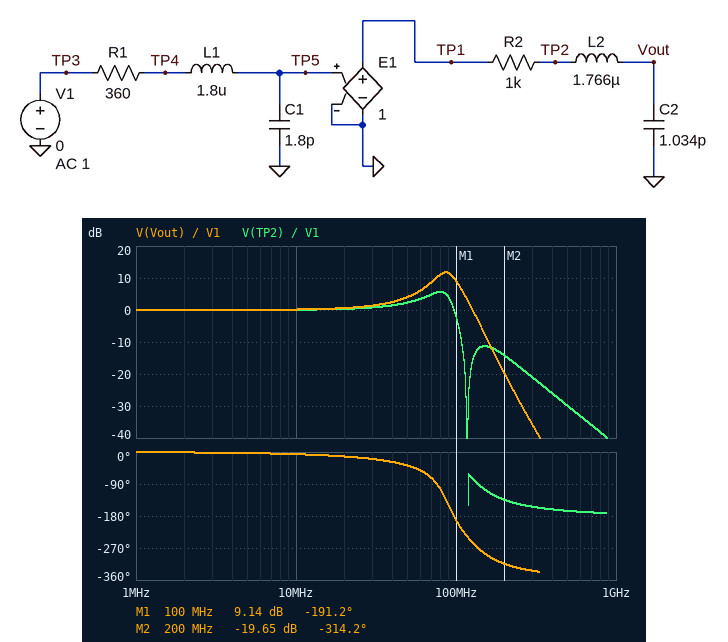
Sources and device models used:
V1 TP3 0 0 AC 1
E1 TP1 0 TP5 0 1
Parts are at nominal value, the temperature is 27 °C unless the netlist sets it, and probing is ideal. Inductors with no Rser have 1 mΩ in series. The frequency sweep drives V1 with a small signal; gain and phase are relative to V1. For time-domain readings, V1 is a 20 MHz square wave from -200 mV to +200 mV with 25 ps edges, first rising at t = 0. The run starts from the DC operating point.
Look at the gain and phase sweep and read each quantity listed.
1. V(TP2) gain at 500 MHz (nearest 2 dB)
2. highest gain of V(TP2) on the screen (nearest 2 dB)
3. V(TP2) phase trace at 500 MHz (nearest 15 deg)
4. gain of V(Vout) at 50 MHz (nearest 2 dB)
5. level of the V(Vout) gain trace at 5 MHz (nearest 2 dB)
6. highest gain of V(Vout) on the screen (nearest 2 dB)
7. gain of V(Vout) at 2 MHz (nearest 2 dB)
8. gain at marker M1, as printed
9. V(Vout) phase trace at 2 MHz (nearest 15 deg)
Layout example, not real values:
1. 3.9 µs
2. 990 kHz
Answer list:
1. -30 dB
2. 6 dB
3. -165 deg
4. 4 dB
5. 0 dB
6. 12 dB
7. 0 dB
8. 9.14 dB
9. 0 deg
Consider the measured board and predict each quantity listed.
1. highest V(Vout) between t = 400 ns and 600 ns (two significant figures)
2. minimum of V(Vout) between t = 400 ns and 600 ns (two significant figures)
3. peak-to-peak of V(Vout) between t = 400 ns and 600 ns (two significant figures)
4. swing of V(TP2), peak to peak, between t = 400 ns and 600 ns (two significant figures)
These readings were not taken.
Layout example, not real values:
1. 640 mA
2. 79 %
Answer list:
1. 510 mV
2. -510 mV
3. 1.0 V
4. 670 mV
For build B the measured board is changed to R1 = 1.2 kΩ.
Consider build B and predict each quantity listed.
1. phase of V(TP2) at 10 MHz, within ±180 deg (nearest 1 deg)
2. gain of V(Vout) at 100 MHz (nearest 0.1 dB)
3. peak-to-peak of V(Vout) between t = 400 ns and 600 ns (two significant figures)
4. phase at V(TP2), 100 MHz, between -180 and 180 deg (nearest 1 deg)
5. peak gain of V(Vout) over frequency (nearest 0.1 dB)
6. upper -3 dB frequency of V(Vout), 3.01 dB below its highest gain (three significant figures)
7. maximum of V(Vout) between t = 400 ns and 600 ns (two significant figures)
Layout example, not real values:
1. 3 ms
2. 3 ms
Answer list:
1. -12 deg
2. 0.2 dB
3. 600 mV
4. -168 deg
5. 1.9 dB
6. 109 MHz
7. 300 mV
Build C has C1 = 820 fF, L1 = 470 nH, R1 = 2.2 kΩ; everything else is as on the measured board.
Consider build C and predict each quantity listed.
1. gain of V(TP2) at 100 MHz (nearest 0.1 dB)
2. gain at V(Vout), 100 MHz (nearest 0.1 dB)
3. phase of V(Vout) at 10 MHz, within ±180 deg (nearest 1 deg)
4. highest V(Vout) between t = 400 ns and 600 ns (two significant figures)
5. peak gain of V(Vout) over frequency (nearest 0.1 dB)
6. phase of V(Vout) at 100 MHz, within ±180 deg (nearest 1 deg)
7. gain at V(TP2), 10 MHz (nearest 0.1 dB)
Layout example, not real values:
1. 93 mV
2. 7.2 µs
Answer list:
1. -11.1 dB
2. 0 dB
3. -10 deg
4. 250 mV
5. 0.4 dB
6. -120 deg
7. -0.1 dB
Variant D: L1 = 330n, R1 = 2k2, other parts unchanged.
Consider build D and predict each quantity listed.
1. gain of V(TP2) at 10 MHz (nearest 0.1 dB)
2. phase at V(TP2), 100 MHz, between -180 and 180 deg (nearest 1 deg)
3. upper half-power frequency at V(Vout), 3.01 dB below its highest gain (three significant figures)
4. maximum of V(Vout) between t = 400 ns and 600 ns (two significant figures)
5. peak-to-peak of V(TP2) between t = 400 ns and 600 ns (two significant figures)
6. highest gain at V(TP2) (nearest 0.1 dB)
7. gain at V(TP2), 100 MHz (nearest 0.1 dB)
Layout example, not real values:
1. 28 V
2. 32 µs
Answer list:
1. -0.3 dB
2. -140 deg
3. 54.1 MHz
4. 200 mV
5. 400 mV
6. 0 dB
7. -16.4 dB
